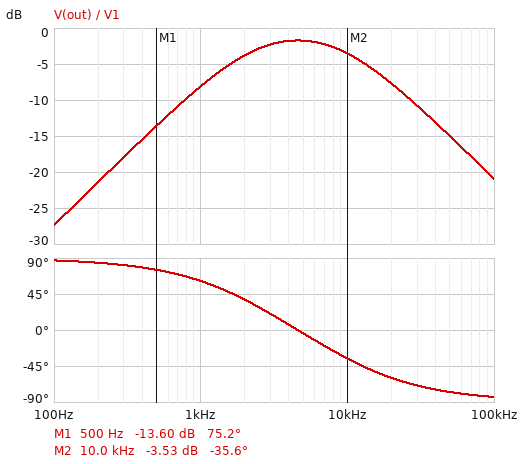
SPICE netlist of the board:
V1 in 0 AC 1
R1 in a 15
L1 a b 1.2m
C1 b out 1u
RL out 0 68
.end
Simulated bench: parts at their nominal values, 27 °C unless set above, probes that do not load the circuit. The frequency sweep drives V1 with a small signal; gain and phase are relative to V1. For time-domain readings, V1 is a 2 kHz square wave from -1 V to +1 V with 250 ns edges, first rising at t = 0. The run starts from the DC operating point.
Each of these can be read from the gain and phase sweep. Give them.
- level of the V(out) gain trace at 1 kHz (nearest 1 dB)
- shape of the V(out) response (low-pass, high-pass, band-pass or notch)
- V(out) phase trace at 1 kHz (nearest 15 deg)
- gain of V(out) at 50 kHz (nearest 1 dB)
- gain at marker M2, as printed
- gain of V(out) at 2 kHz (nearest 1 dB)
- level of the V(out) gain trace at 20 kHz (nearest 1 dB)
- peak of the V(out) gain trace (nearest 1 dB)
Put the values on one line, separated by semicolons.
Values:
-8 dB; band-pass; 60 deg; -15 dB; -3.53 dB; -4 dB; -8 dB; -2 dB
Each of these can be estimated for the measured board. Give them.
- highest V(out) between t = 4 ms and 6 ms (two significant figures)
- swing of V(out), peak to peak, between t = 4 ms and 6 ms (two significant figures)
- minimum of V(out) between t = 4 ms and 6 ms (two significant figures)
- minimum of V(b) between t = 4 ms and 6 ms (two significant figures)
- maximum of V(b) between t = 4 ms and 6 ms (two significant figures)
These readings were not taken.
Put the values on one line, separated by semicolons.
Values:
1.2 V; 2.5 V; -1.2 V; -1.0 V; 1.0 V
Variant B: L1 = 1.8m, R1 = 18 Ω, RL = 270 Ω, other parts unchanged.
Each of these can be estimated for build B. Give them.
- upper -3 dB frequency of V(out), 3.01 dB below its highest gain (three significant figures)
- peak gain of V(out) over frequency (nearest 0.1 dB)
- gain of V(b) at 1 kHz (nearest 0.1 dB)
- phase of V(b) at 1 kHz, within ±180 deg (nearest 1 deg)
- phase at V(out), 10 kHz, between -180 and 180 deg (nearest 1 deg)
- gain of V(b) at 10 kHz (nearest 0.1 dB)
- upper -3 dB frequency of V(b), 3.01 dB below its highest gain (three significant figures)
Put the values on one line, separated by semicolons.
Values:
26.0 kHz; -0.6 dB; -0.3 dB; -3 deg; -19 deg; -1.0 dB; 22.8 kHz
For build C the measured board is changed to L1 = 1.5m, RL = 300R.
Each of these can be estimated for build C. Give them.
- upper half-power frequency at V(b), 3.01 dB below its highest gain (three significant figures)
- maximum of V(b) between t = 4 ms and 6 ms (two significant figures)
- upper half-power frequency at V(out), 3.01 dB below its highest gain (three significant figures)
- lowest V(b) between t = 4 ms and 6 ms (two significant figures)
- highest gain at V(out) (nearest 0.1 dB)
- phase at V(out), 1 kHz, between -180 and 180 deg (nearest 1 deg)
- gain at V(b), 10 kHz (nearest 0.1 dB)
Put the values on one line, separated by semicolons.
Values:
30.7 kHz; 980 mV; 33.9 kHz; -980 mV; -0.4 dB; 25 deg; -0.7 dB
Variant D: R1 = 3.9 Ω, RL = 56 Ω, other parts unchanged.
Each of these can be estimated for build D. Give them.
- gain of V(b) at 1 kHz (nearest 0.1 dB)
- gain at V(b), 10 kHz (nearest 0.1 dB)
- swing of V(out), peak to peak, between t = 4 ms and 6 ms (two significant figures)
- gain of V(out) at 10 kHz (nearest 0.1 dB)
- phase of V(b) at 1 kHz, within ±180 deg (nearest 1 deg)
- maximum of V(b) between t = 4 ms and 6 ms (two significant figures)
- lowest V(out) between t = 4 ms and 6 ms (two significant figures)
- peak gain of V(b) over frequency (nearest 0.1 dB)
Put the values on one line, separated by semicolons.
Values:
0.3 dB; -3.2 dB; 2.6 V; -3.6 dB; -2 deg; 1.3 V; -1.3 V; 1.2 dB
